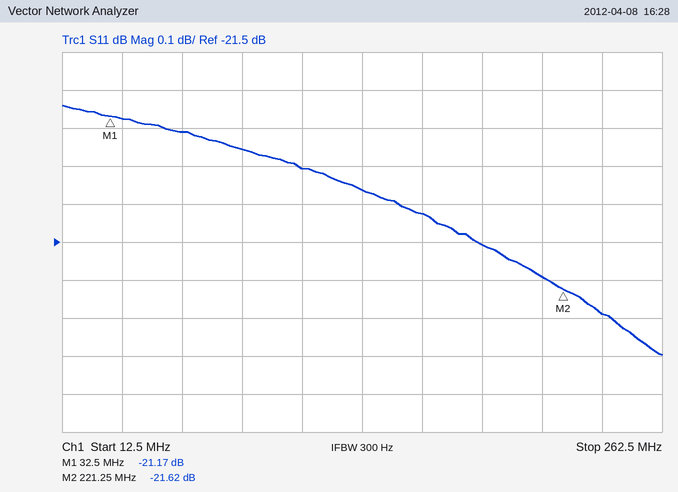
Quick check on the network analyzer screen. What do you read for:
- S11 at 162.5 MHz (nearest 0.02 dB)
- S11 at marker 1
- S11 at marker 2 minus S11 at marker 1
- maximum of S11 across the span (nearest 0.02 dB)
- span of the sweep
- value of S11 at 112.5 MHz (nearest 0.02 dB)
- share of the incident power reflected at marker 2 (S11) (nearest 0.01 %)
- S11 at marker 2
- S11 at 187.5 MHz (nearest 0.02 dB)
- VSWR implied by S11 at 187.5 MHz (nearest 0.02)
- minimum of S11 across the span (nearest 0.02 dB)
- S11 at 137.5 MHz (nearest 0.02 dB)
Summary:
-21.42 dB
-21.17 dB
-0.45 dB
-21.14 dB
250 MHz
-21.30 dB
0.69 %
-21.62 dB
-21.50 dB
1.18
-21.80 dB
-21.36 dB
